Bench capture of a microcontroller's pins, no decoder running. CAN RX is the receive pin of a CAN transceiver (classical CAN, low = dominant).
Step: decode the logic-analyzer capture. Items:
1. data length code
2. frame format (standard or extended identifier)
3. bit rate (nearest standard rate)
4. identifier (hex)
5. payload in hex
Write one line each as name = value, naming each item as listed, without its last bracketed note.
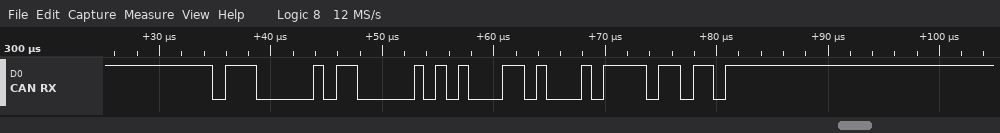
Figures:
data length code = 1
frame format = standard
bit rate = 1000 kbit/s
identifier = 0x703
payload in hex = 46
